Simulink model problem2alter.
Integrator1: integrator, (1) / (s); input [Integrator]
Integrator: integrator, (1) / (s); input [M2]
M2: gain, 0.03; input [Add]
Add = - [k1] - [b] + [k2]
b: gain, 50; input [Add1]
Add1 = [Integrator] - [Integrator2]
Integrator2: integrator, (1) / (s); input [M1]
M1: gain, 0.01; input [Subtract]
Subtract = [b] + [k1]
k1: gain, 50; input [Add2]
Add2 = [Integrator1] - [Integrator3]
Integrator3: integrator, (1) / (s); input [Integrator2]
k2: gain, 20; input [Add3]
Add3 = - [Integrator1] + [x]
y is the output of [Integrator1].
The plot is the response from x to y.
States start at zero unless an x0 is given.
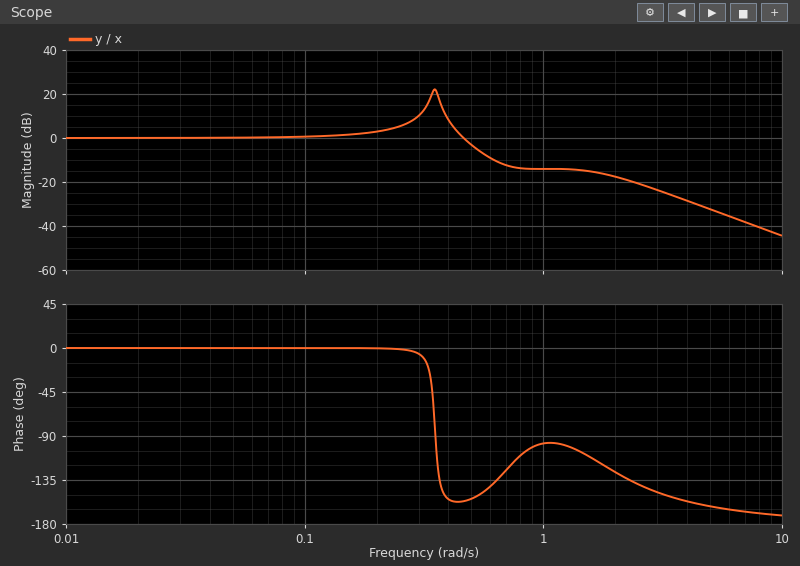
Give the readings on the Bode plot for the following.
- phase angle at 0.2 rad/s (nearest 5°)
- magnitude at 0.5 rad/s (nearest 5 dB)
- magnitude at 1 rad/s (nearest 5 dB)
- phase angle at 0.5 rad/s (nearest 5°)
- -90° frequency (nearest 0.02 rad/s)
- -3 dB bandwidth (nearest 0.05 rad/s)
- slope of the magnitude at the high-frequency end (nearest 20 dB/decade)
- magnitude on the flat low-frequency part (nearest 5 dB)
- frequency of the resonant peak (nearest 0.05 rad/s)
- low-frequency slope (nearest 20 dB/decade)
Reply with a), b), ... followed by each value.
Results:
a) 0°
b) -5 dB
c) -15 dB
d) -155°
e) 0.36 rad/s
f) 0.50 rad/s
g) -40 dB/decade
h) 0 dB
i) 0.35 rad/s
j) 0 dB/decade
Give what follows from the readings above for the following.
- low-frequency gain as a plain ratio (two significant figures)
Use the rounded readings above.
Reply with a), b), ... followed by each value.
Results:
a) 1.0
